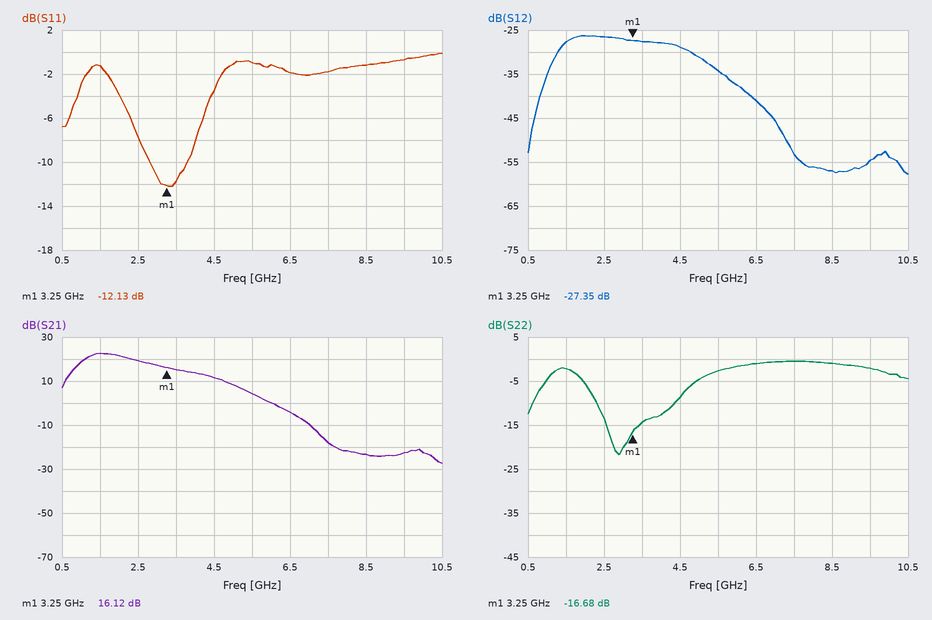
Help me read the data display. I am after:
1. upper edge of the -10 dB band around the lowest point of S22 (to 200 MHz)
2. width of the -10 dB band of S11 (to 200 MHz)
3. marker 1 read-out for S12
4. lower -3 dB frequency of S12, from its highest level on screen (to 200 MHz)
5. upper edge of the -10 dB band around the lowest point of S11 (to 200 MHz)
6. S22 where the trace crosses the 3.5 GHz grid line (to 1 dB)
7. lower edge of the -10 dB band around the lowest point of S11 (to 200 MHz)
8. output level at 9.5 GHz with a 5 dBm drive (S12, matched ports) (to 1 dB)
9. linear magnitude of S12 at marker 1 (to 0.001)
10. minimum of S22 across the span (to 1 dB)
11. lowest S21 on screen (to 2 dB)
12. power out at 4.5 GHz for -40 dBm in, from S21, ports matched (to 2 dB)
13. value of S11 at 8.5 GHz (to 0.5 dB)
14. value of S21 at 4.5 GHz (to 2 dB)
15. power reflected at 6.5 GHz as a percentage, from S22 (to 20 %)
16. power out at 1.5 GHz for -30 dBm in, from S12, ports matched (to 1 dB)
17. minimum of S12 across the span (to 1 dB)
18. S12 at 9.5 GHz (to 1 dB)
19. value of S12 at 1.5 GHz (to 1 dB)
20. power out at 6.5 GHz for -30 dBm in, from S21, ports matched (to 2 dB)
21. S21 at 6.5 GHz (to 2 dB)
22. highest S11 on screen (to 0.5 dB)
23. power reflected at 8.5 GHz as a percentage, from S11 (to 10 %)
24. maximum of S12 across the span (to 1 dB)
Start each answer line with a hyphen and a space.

- 4.4 GHz
- 1.0 GHz
- -27.35 dB
- 1.4 GHz
- 3.8 GHz
- -14 dB
- 2.8 GHz
- -50 dBm
- 0.043
- -22 dB
- -28 dB
- -28 dBm
- -1.0 dB
- 12 dB
- 80 %
- -58 dBm
- -58 dB
- -55 dB
- -28 dB
- -34 dBm
- -4 dB
- 0.0 dB
- 80 %
- -26 dB
